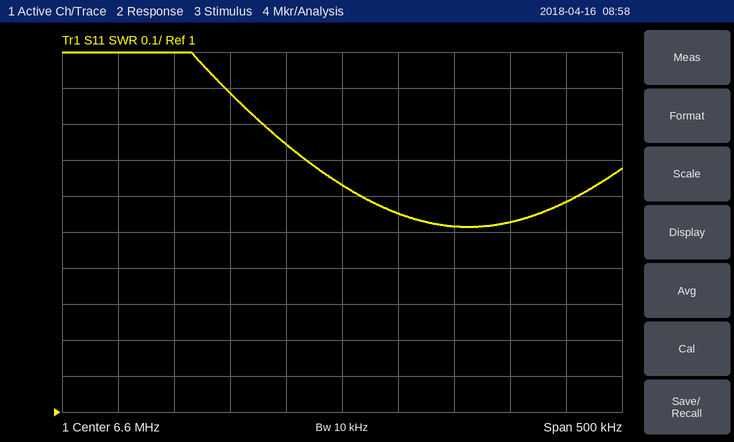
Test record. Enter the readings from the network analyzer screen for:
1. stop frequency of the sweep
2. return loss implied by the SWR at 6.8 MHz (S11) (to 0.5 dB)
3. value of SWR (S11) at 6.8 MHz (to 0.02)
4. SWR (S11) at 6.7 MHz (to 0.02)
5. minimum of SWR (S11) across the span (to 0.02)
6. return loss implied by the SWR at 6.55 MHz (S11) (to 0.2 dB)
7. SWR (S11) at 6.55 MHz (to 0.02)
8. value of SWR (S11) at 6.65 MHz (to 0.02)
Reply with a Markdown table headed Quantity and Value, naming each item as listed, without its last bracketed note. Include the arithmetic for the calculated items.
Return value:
| Quantity | Value |
|---|---|
| stop frequency of the sweep | 6.85 MHz |
| return loss implied by the SWR at 6.8 MHz (S11) | −20 log10((1.58 − 1)/(1.58 + 1)) ≈ 13.0 dB |
| value of SWR (S11) at 6.8 MHz | 1.58 |
| SWR (S11) at 6.7 MHz | 1.52 |
| minimum of SWR (S11) across the span | 1.52 |
| return loss implied by the SWR at 6.55 MHz (S11) | −20 log10((1.74 − 1)/(1.74 + 1)) ≈ 11.4 dB |
| SWR (S11) at 6.55 MHz | 1.74 |
| value of SWR (S11) at 6.65 MHz | 1.56 |
